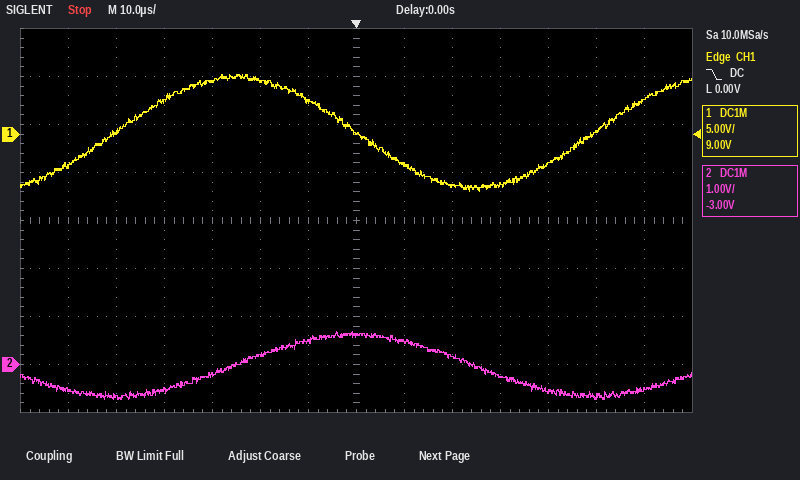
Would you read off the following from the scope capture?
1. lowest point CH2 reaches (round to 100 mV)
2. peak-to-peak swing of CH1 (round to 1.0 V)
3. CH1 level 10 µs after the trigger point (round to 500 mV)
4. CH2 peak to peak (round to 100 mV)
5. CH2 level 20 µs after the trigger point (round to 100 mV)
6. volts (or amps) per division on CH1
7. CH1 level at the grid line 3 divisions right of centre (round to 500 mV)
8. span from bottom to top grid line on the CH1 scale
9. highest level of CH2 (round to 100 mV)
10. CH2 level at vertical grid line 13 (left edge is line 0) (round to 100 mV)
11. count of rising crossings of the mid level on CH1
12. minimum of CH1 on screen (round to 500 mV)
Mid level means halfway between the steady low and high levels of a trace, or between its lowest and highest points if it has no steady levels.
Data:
-700 mV
12.0 V
-3.0 V
1.4 V
200 mV
5 V
-5.5 V
40 V
700 mV
-500 mV
2
-6.0 V
